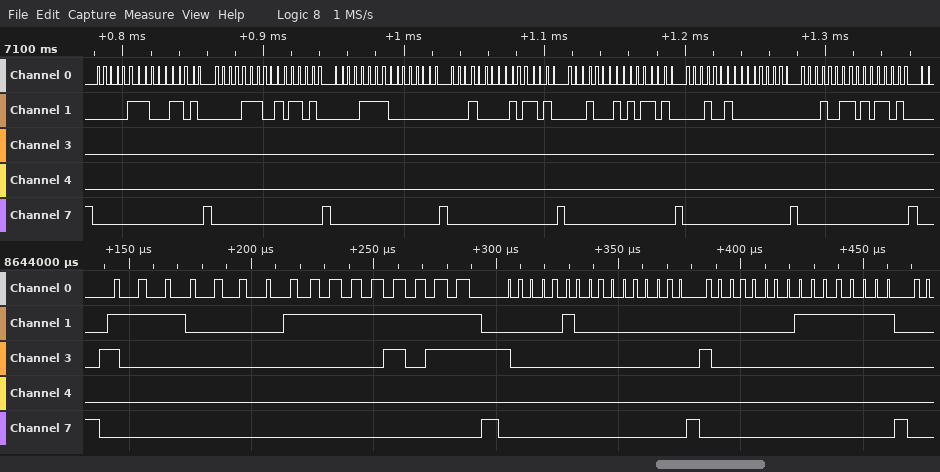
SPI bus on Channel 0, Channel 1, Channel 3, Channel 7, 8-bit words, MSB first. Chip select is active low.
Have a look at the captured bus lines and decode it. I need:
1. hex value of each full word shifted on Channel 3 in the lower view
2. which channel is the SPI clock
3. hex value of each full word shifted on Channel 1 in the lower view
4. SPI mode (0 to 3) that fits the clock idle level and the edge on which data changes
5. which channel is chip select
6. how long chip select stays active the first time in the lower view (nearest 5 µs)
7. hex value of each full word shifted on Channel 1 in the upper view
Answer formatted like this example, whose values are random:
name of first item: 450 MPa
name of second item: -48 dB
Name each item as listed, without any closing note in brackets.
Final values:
hex value of each full word shifted on Channel 3 in the lower view: 80, 0B, 80, 00, 80, 00
which channel is the SPI clock: Channel 0
hex value of each full word shifted on Channel 1 in the lower view: E1, FF, 04, 00, 00, FF
SPI mode (0 to 3) that fits the clock idle level and the edge on which data changes: 0
which channel is chip select: Channel 7
how long chip select stays active the first time in the lower view: 155 µs
hex value of each full word shifted on Channel 1 in the upper view: 07, 1A, 0E, 5A, 0F, 00, 10, 5A, 11, 5A, 12, 00, 13, 5A
